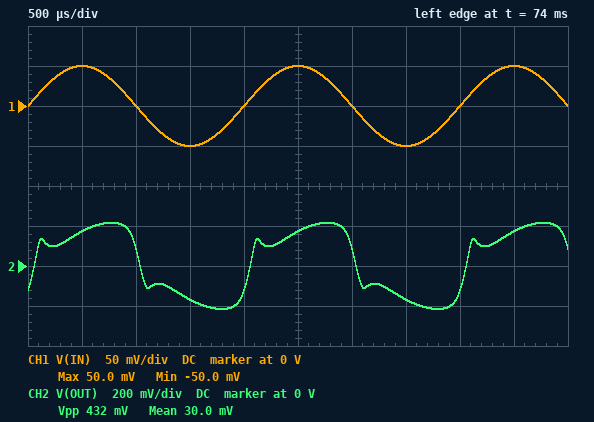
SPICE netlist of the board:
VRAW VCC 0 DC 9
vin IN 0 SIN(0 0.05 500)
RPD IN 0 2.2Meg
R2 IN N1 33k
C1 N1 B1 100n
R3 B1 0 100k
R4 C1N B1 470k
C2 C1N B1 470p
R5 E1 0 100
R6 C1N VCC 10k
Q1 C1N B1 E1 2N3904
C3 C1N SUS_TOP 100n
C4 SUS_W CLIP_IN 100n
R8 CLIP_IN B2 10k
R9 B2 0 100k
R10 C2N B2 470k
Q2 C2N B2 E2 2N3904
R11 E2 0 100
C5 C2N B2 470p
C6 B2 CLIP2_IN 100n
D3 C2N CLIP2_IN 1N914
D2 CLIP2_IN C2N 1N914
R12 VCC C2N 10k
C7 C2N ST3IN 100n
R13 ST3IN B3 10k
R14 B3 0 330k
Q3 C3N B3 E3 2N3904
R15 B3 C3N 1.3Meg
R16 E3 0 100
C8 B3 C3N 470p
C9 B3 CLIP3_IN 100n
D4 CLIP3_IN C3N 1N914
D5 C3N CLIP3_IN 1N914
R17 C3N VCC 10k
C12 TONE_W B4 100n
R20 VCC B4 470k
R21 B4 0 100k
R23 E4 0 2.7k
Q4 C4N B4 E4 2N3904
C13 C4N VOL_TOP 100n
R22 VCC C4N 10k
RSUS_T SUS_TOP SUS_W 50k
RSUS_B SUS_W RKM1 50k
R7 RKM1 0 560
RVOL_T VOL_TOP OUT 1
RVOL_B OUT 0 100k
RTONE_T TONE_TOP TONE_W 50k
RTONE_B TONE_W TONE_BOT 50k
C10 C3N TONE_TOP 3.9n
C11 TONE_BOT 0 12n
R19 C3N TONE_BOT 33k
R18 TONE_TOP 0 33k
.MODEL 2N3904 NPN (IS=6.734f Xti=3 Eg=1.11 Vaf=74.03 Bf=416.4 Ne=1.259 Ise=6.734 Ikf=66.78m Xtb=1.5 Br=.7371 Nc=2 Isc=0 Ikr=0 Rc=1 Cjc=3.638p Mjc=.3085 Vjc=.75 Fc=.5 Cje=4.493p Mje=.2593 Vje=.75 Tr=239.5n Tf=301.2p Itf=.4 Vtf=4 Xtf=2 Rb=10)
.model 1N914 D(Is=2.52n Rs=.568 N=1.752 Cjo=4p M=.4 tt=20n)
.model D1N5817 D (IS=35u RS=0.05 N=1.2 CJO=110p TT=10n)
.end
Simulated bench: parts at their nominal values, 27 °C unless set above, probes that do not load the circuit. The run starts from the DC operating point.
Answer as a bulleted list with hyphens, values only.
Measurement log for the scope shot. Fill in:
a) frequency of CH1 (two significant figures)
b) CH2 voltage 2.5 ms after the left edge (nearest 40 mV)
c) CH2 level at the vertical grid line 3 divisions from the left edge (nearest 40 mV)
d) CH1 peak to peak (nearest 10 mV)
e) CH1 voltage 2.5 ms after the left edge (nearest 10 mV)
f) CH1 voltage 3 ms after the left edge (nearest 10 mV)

- 500 Hz
- 160 mV
- -160 mV
- 100 mV
- 50 mV
- 0 V
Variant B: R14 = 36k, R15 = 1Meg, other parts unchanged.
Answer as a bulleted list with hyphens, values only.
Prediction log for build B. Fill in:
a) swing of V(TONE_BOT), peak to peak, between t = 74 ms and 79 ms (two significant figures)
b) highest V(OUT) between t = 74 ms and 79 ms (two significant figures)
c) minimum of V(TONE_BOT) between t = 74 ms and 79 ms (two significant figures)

- 3.1 mV
- 1.2 mV
- 6.7 V
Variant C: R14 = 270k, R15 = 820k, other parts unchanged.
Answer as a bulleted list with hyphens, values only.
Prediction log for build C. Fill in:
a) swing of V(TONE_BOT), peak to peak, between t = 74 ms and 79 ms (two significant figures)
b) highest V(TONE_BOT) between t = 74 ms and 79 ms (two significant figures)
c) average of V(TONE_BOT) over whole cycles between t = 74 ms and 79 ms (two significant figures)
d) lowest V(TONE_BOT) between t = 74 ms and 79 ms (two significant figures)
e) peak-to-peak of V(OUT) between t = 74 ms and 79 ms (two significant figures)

- 470 mV
- 6.1 V
- 5.9 V
- 5.6 V
- 450 mV
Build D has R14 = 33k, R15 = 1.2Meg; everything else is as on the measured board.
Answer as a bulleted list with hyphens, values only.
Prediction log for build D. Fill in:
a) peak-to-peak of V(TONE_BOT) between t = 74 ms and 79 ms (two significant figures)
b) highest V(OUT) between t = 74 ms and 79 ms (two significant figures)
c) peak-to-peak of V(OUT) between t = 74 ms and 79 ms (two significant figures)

- 3.1 mV
- 1.4 mV
- 2.8 mV
